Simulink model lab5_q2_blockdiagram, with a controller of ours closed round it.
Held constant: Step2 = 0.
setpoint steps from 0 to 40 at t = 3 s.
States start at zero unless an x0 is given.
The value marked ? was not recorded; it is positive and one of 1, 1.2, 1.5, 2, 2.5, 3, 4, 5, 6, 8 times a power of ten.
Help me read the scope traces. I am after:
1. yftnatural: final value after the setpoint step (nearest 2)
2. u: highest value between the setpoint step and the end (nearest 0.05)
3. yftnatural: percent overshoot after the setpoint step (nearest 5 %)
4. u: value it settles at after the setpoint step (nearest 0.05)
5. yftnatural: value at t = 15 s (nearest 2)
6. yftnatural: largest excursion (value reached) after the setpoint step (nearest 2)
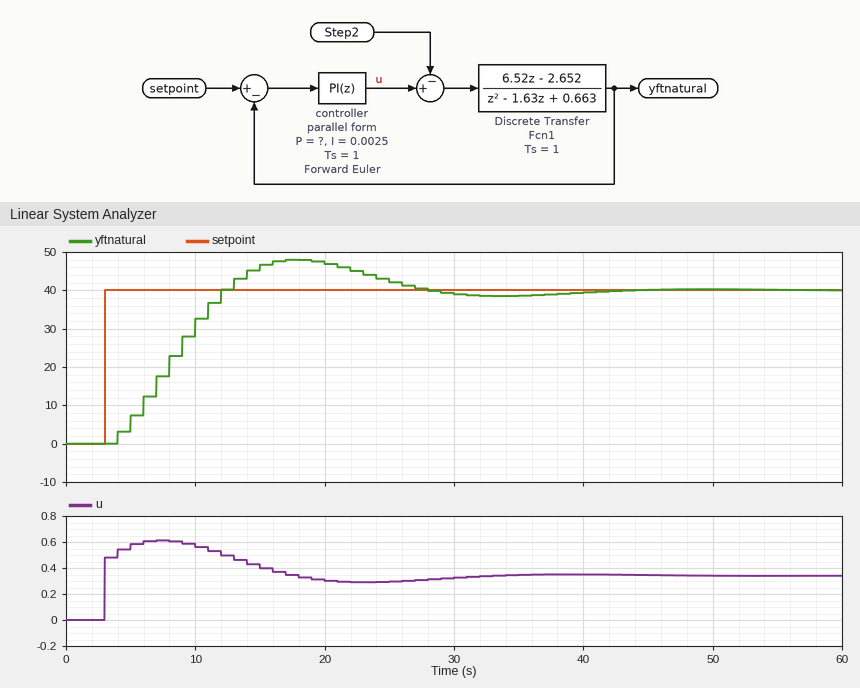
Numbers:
40
0.60
20 %
0.35
46
48
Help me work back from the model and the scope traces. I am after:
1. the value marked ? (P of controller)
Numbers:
0.012
